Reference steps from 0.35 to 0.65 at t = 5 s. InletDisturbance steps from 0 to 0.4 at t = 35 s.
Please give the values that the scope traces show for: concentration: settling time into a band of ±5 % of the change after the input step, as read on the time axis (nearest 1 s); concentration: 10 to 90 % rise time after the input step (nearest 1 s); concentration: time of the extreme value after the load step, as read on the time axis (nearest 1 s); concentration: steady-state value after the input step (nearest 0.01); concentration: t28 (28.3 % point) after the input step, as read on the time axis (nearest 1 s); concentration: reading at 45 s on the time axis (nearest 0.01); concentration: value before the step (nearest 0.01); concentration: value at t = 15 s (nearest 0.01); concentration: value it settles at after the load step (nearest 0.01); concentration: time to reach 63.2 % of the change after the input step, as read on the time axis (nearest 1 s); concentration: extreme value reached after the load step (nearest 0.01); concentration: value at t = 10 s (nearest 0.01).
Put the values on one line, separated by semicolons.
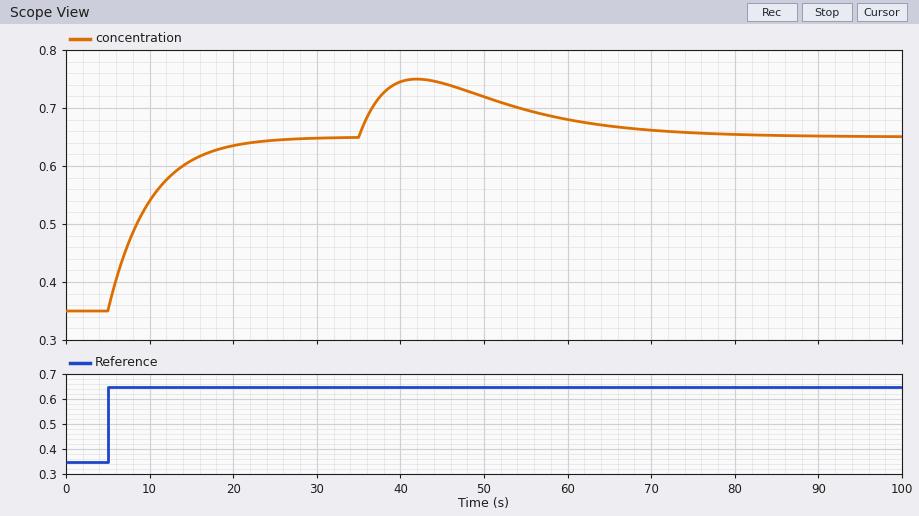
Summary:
20 s; 11 s; 42 s; 0.65; 7 s; 0.74; 0.35; 0.61; 0.65; 10 s; 0.75; 0.54
